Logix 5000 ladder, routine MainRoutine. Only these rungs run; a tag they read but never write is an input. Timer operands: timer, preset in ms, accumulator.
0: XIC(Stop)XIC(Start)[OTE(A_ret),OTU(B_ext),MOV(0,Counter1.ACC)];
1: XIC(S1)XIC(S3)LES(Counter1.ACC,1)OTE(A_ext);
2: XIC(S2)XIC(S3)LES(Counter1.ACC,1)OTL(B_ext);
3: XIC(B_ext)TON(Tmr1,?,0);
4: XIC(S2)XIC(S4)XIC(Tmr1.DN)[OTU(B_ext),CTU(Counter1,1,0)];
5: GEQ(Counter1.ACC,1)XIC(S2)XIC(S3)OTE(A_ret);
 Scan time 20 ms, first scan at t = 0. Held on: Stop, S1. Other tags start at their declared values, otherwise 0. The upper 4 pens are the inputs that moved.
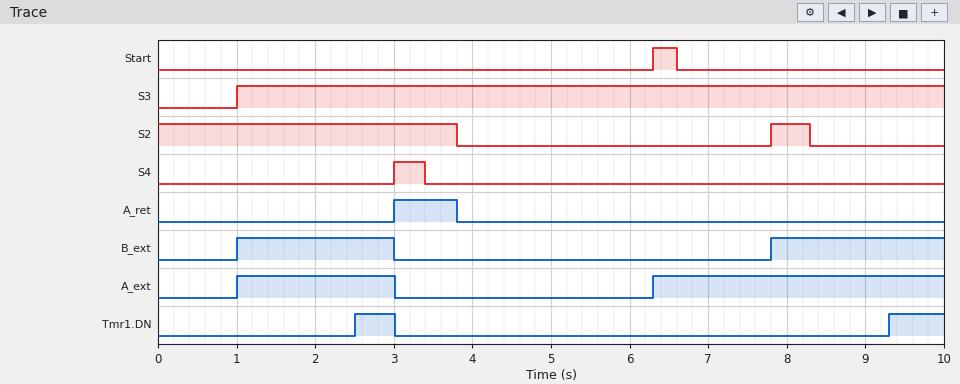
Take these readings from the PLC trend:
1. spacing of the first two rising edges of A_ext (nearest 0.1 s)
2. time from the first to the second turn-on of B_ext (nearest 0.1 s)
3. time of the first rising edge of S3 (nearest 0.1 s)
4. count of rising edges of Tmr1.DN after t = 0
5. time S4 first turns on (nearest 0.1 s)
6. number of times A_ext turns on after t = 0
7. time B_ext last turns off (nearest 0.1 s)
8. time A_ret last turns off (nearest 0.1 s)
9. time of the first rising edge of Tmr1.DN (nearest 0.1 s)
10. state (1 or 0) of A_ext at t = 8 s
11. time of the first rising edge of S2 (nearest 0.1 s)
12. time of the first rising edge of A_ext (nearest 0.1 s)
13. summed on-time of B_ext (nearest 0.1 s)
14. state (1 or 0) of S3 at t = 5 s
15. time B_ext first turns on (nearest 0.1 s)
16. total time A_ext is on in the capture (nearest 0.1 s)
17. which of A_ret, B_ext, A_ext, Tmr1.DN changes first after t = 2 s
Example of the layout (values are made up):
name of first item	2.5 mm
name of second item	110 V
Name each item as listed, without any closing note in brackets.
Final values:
spacing of the first two rising edges of A_ext	5.3 s
time from the first to the second turn-on of B_ext	6.8 s
time of the first rising edge of S3	1.0 s
count of rising edges of Tmr1.DN after t = 0	2
time S4 first turns on	3.0 s
number of times A_ext turns on after t = 0	2
time B_ext last turns off	3.0 s
time A_ret last turns off	3.8 s
time of the first rising edge of Tmr1.DN	2.5 s
state (1 or 0) of A_ext at t = 8 s	1
time of the first rising edge of S2	7.8 s
time of the first rising edge of A_ext	1.0 s
summed on-time of B_ext	4.2 s
state (1 or 0) of S3 at t = 5 s	1
time B_ext first turns on	1.0 s
total time A_ext is on in the capture	5.7 s
which of A_ret, B_ext, A_ext, Tmr1.DN changes first after t = 2 s	Tmr1.DN
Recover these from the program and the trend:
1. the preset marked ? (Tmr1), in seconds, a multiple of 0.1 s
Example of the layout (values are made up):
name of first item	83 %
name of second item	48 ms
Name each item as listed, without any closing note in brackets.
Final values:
the preset marked ? (Tmr1), in seconds, a multiple of 0.1 s	1.5 s
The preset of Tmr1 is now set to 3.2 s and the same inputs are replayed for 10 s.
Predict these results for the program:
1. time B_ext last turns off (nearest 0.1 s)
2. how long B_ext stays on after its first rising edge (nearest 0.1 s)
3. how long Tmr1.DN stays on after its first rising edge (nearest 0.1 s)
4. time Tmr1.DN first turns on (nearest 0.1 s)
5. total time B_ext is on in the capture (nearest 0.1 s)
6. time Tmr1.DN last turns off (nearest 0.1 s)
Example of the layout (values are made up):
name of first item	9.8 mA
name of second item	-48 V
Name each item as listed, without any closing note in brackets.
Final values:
time B_ext last turns off	6.3 s
how long B_ext stays on after its first rising edge	5.3 s
how long Tmr1.DN stays on after its first rising edge	2.1 s
time Tmr1.DN first turns on	4.2 s
total time B_ext is on in the capture	7.5 s
time Tmr1.DN last turns off	6.3 s
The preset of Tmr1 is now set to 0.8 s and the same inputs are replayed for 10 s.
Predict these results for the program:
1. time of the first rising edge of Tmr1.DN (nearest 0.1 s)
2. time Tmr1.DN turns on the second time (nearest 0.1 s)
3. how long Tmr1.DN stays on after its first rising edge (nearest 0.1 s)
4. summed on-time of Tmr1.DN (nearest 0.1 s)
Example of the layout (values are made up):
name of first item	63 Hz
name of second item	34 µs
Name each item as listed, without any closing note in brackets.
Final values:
time of the first rising edge of Tmr1.DN	1.8 s
time Tmr1.DN turns on the second time	8.6 s
how long Tmr1.DN stays on after its first rising edge	1.2 s
summed on-time of Tmr1.DN	2.6 s
